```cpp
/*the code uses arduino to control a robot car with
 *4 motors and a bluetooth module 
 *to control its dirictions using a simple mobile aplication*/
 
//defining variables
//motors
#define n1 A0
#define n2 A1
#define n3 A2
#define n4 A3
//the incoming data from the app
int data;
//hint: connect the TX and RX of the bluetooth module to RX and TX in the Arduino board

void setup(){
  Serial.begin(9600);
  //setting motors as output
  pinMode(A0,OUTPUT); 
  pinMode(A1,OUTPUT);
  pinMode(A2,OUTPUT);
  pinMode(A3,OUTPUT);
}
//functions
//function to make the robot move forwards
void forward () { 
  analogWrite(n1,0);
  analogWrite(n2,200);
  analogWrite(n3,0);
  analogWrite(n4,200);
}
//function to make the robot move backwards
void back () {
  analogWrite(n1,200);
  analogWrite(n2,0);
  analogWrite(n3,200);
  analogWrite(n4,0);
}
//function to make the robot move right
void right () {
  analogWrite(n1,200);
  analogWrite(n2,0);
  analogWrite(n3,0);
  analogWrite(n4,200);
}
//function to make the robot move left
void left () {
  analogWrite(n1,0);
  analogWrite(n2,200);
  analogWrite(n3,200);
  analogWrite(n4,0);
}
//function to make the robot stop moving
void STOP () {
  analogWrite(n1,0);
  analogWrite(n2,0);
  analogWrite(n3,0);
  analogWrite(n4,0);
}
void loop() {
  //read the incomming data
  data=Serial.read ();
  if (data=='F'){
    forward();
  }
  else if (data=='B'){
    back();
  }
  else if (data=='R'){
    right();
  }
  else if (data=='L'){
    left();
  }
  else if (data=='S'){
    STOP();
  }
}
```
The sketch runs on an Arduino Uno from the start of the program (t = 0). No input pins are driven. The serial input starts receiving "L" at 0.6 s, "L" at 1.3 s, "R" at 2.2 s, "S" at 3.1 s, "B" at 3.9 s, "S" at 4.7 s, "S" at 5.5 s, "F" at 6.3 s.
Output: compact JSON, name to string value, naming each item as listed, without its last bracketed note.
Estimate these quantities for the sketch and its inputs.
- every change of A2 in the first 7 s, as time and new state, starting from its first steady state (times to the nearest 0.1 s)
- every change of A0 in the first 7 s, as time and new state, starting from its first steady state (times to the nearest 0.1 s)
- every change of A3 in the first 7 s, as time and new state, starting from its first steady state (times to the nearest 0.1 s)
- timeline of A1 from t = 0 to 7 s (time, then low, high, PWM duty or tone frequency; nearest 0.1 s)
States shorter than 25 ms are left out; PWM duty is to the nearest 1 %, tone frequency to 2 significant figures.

{"every change of A2 in the first 7 s, as time and new state, starting from its first steady state": "0 s low; 0.6 s high; 2.2 s low; 3.9 s high; 4.7 s low", "every change of A0 in the first 7 s, as time and new state, starting from its first steady state": "0 s low; 2.2 s high; 3.1 s low; 3.9 s high; 4.7 s low", "every change of A3 in the first 7 s, as time and new state, starting from its first steady state": "0 s low; 2.2 s high; 3.1 s low; 6.3 s high", "timeline of A1 from t = 0 to 7 s": "0 s low; 0.6 s high; 2.2 s low; 6.3 s high"}
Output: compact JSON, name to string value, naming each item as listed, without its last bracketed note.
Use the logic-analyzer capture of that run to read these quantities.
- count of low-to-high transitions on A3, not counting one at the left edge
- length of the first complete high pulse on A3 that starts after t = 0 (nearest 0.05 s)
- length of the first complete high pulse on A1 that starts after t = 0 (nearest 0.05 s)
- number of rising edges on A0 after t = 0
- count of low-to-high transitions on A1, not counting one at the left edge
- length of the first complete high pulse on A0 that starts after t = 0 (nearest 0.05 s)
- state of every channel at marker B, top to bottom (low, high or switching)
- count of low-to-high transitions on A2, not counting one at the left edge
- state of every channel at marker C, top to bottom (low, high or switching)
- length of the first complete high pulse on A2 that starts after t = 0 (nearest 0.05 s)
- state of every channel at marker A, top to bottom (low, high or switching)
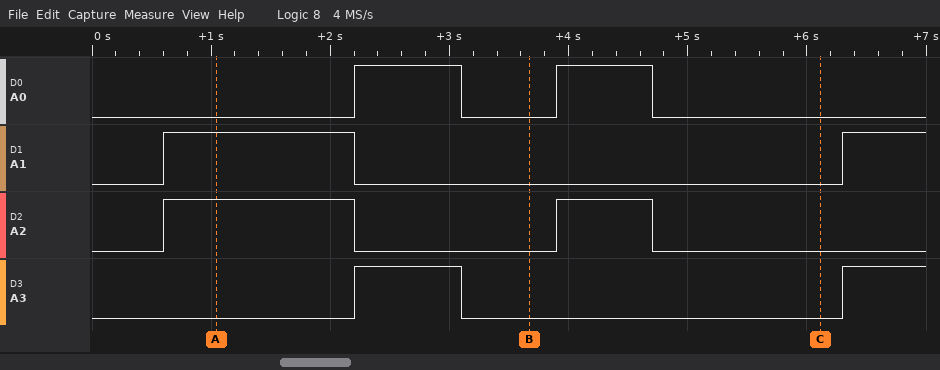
{"count of low-to-high transitions on A3, not counting one at the left edge": "2", "length of the first complete high pulse on A3 that starts after t = 0": "0.90 s", "length of the first complete high pulse on A1 that starts after t = 0": "1.60 s", "number of rising edges on A0 after t = 0": "2", "count of low-to-high transitions on A1, not counting one at the left edge": "2", "length of the first complete high pulse on A0 that starts after t = 0": "0.90 s", "state of every channel at marker B, top to bottom": "A0 low, A1 low, A2 low, A3 low", "count of low-to-high transitions on A2, not counting one at the left edge": "2", "state of every channel at marker C, top to bottom": "A0 low, A1 low, A2 low, A3 low", "length of the first complete high pulse on A2 that starts after t = 0": "1.60 s", "state of every channel at marker A, top to bottom": "A0 low, A1 high, A2 high, A3 low"}
